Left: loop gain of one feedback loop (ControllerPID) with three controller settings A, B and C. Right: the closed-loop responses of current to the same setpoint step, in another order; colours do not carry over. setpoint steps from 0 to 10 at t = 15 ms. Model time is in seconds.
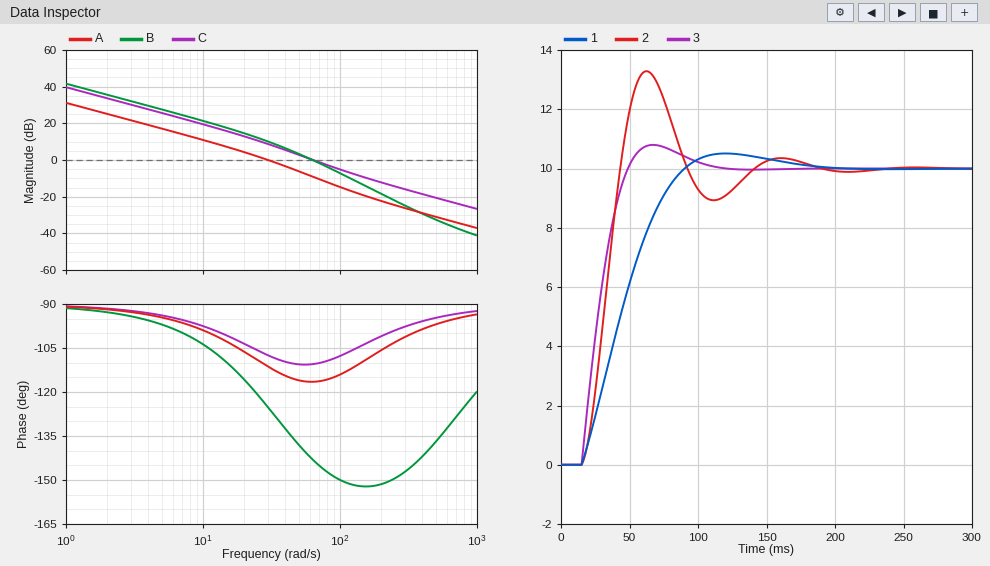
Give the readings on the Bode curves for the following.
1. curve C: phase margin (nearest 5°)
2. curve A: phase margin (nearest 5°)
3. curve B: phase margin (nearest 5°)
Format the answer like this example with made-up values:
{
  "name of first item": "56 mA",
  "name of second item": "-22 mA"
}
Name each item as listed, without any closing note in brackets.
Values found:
{
  "curve C: phase margin": "70°",
  "curve A: phase margin": "70°",
  "curve B: phase margin": "35°"
}
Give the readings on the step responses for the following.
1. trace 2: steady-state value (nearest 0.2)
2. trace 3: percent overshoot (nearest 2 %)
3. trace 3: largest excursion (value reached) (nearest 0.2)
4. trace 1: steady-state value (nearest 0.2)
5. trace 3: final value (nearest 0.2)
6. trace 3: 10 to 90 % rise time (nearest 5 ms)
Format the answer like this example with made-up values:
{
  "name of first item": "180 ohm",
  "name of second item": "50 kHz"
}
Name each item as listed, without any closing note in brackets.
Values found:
{
  "trace 2: steady-state value": "10.0",
  "trace 3: percent overshoot": "8 %",
  "trace 3: largest excursion (value reached)": "10.8",
  "trace 1: steady-state value": "10.0",
  "trace 3: final value": "10.0",
  "trace 3: 10 to 90 % rise time": "25 ms"
}
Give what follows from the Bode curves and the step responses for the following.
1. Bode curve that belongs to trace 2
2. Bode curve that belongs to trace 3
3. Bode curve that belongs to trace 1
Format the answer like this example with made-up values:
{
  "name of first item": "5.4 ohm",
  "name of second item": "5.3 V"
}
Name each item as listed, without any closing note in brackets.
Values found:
{
  "Bode curve that belongs to trace 2": "B",
  "Bode curve that belongs to trace 3": "C",
  "Bode curve that belongs to trace 1": "A"
}
